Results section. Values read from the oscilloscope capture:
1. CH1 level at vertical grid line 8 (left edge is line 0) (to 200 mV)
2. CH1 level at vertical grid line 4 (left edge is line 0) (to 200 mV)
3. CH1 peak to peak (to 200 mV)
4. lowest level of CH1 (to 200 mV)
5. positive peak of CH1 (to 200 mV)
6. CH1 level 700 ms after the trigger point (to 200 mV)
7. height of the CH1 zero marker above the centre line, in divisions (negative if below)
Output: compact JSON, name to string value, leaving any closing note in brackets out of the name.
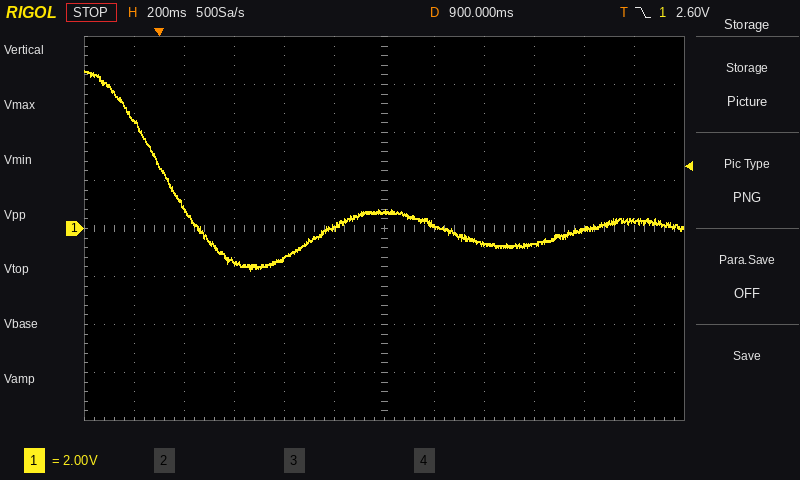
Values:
{"CH1 level at vertical grid line 8 (left edge is line 0)": "-600 mV", "CH1 level at vertical grid line 4 (left edge is line 0)": "-1.2 V", "CH1 peak to peak": "8.4 V", "lowest level of CH1": "-1.8 V", "positive peak of CH1": "6.6 V", "CH1 level 700 ms after the trigger point": "0.0 V", "height of the CH1 zero marker above the centre line, in divisions": "0.0 div"}
